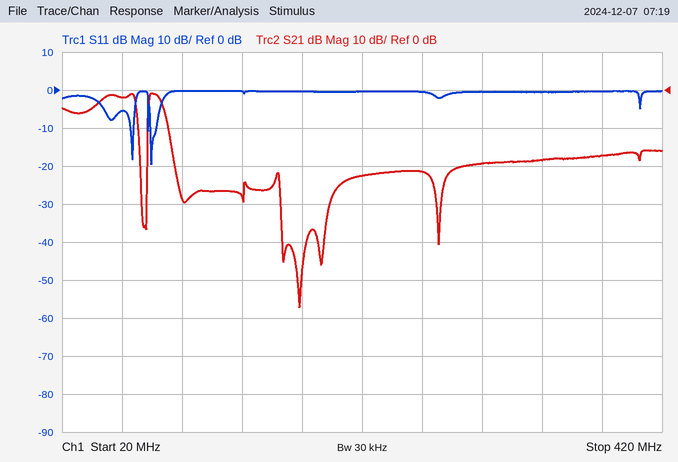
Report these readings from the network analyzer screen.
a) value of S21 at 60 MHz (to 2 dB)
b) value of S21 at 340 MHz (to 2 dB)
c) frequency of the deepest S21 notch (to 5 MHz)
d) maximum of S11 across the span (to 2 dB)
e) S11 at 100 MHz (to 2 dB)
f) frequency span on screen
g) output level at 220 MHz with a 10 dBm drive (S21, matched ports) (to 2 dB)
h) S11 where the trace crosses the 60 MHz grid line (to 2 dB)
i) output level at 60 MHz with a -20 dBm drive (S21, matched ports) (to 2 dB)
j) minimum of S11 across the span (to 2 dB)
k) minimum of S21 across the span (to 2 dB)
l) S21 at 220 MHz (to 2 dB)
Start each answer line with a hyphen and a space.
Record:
- -2 dB
- -18 dB
- 180 MHz
- 0 dB
- 0 dB
- 400 MHz
- -12 dBm
- -6 dB
- -22 dBm
- -20 dB
- -58 dB
- -22 dB
